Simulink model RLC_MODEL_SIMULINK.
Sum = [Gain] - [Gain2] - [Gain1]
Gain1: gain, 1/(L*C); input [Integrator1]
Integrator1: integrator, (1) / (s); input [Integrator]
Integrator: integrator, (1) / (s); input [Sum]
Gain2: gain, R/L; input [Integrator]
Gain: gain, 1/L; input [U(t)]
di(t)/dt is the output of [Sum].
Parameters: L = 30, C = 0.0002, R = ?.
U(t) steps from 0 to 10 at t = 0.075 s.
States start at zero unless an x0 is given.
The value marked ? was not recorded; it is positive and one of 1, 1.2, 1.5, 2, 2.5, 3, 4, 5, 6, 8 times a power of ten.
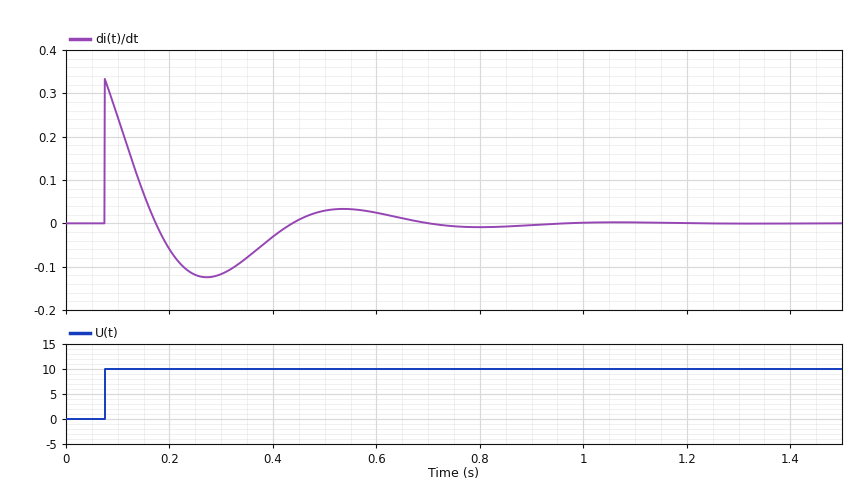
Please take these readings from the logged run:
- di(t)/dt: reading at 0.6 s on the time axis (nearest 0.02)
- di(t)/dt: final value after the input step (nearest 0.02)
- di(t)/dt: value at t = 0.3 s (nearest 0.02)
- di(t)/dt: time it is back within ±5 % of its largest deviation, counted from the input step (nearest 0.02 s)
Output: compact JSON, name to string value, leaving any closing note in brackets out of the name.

{"di(t)/dt: reading at 0.6 s on the time axis": "0.02", "di(t)/dt: final value after the input step": "0.00", "di(t)/dt: value at t = 0.3 s": "-0.12", "di(t)/dt: time it is back within ±5 % of its largest deviation, counted from the input step": "0.56 s"}
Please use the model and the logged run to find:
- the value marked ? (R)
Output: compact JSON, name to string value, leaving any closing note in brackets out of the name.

{"the value marked ?": "300"}
